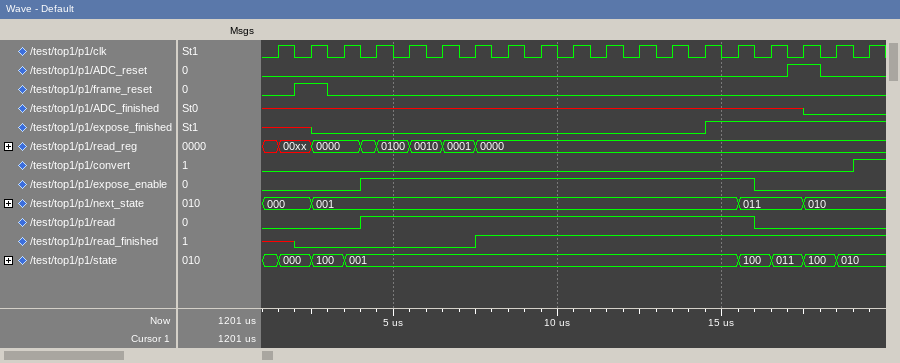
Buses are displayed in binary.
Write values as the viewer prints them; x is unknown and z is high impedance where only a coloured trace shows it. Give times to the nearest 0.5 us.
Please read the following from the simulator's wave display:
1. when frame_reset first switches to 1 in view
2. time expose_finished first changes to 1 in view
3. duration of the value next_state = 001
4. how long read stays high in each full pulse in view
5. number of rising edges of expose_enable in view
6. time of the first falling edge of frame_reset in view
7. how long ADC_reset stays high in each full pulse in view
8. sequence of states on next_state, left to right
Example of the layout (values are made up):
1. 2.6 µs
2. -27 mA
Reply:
1. 2 us
2. 14.5 us
3. 13 us
4. 12 us
5. 1
6. 3 us
7. 1 us
8. 000, 001, 011, 010
